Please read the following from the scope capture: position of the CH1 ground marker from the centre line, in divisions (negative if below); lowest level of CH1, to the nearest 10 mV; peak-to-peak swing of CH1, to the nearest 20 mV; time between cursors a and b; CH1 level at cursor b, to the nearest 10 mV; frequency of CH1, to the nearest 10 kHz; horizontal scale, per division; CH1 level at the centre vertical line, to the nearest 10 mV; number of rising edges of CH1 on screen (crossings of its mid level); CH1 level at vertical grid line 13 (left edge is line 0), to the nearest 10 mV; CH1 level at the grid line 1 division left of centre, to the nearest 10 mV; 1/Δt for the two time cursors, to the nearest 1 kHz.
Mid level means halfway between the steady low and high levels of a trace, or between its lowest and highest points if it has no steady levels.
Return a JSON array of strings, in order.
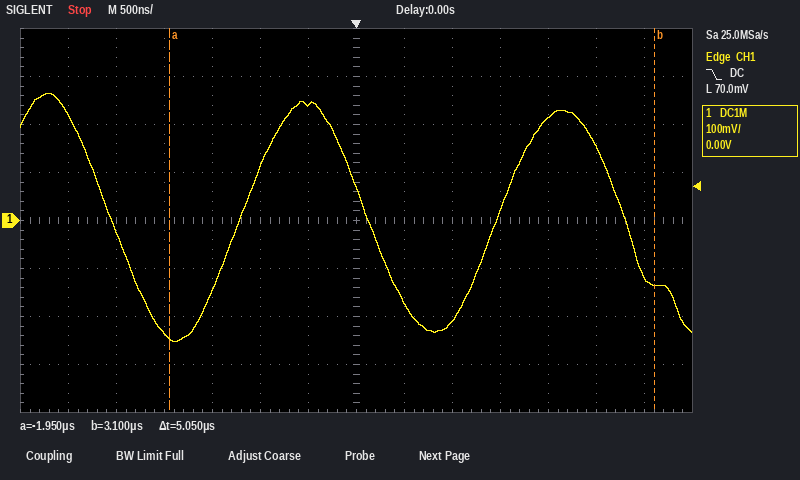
["0.0 div", "-250 mV", "520 mV", "5.05 µs", "-130 mV", "370 kHz", "500 ns", "70 mV", "2", "-120 mV", "240 mV", "198 kHz"]
